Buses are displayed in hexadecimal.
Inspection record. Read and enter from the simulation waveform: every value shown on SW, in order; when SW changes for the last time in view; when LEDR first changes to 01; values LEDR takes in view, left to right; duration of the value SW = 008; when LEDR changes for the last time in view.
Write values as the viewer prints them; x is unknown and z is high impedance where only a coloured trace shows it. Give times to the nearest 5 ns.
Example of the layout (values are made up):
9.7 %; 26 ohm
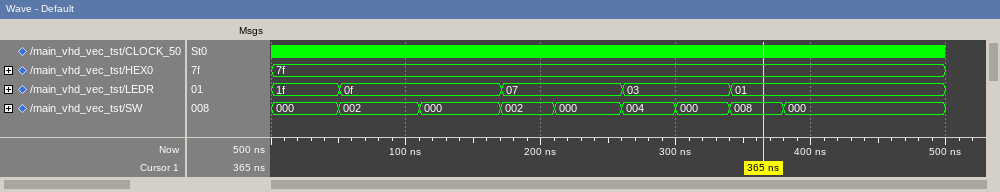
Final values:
000, 002, 000, 002, 000, 004, 000, 008, 000; 380 ns; 340 ns; 1f, 0f, 07, 03, 01; 40 ns; 340 ns
